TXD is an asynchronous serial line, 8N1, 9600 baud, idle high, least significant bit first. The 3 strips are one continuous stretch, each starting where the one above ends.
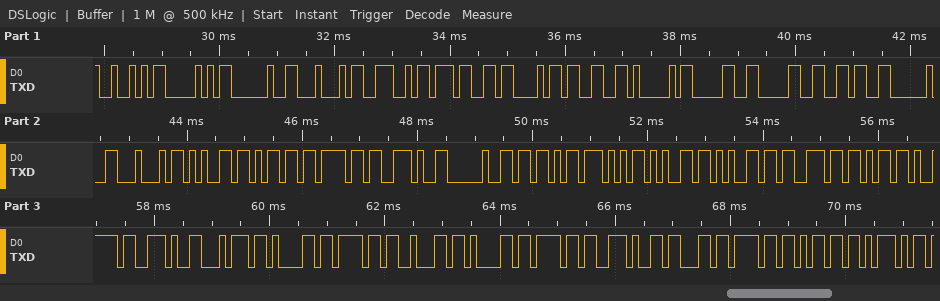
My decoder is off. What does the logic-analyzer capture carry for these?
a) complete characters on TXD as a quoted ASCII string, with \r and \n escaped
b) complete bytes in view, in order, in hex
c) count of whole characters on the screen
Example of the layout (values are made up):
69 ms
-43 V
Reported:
"RP DN7C3A006 Demo. [Weesky.taobao.com]"
0x52 0x50 0x20 0x44 0x4E 0x37 0x43 0x33 0x41 0x30 0x30 0x36 0x20 0x44 0x65 0x6D 0x6F 0x2E 0x20 0x5B 0x57 0x65 0x65 0x73 0x6B 0x79 0x2E 0x74 0x61 0x6F 0x62 0x61 0x6F 0x2E 0x63 0x6F 0x6D 0x5D
38
